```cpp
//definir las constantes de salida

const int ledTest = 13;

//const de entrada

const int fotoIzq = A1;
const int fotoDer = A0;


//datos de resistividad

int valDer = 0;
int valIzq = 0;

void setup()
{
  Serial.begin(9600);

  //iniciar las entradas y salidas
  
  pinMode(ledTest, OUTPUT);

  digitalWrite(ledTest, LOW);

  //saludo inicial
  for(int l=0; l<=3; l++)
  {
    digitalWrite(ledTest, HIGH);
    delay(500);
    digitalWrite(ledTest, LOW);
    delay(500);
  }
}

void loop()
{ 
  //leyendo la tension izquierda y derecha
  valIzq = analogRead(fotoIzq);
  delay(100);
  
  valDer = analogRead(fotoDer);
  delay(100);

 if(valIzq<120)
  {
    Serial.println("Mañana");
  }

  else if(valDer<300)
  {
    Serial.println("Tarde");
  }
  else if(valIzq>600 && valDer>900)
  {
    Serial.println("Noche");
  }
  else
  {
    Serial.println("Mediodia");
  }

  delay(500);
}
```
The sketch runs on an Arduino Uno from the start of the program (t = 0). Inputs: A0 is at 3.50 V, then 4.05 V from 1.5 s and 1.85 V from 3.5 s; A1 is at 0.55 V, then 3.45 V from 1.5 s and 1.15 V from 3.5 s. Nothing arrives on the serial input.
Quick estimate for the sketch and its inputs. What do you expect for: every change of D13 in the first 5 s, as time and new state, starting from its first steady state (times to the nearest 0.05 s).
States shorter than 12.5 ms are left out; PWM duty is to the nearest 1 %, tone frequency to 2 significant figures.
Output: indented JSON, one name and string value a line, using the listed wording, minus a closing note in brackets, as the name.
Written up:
{
  "every change of D13 in the first 5 s, as time and new state, starting from its first steady state": "0 s high; 0.5 s low; 1 s high; 1.5 s low; 2 s high; 2.5 s low; 3 s high; 3.5 s low"
}
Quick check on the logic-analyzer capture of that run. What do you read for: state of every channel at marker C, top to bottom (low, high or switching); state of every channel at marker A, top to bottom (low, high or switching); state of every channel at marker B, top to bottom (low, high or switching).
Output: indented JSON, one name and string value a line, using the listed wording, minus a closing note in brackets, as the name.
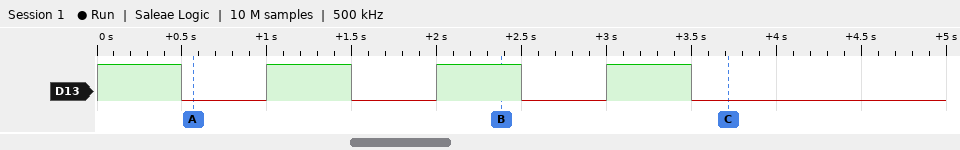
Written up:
{
  "state of every channel at marker C, top to bottom": "D13 low",
  "state of every channel at marker A, top to bottom": "D13 low",
  "state of every channel at marker B, top to bottom": "D13 high"
}
